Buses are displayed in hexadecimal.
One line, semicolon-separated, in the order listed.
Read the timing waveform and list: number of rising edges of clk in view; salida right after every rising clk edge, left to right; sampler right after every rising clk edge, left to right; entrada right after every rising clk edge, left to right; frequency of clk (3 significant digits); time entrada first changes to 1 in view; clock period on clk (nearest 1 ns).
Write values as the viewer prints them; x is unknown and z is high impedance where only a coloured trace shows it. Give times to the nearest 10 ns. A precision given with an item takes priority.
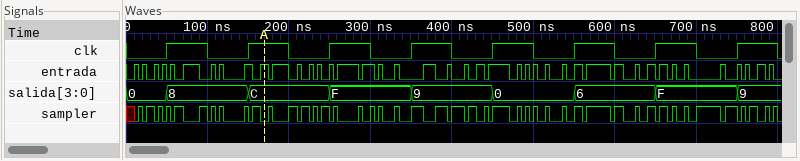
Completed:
8; 8, C, F, 9, 0, 6, F, 9; 1 0 0 1 1 1 0 0; 0 1 1 0 1 1 0 1; 10.0 MHz; 10 ns; 100 ns
